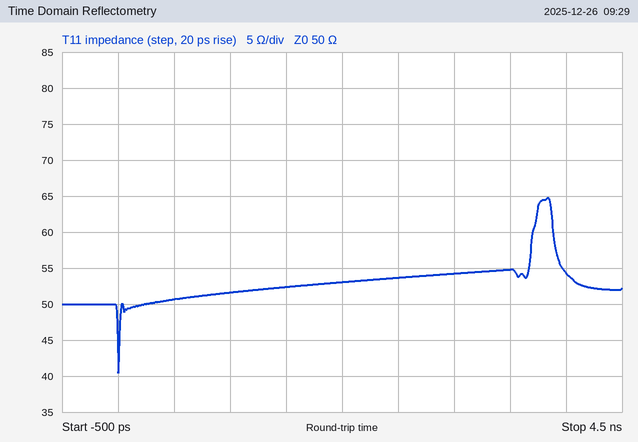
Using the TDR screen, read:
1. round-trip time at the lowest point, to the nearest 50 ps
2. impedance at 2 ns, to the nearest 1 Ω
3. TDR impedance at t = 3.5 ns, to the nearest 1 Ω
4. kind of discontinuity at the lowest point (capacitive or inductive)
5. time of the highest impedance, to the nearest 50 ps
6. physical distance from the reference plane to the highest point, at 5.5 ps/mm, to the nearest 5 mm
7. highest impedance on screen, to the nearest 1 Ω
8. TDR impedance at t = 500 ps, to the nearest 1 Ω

0 ps
53 Ω
55 Ω
capacitive
3.85 ns
350 mm
65 Ω
51 Ω
